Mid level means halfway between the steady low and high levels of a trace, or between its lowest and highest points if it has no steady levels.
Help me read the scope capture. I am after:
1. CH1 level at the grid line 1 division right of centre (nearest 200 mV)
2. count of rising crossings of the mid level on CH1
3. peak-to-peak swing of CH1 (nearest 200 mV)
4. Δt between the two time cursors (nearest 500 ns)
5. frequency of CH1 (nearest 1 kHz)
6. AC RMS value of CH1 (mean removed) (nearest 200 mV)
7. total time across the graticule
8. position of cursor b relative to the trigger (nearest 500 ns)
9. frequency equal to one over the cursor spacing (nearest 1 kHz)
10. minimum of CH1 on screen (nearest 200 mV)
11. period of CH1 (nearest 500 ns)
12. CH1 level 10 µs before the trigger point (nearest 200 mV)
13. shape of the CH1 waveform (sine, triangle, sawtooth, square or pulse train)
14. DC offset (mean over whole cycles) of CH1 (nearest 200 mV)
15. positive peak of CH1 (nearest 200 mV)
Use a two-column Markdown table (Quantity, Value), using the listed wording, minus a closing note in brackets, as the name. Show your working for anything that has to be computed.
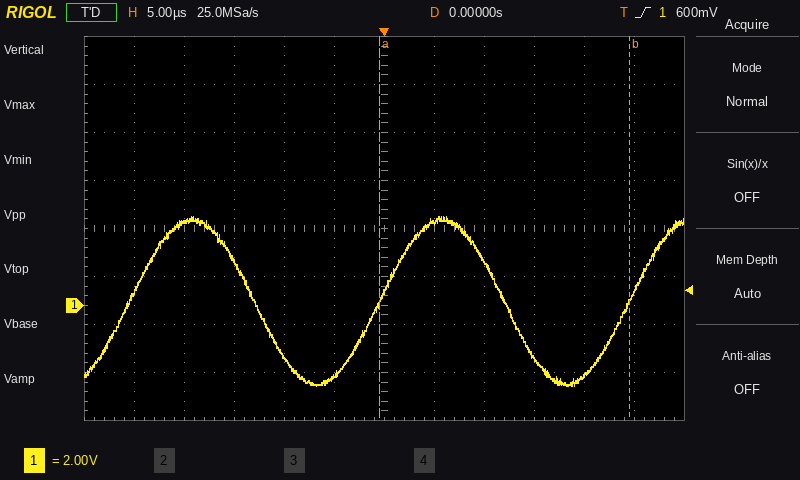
| Quantity | Value |
|---|---|
| CH1 level at the grid line 1 division right of centre | 3.4 V |
| count of rising crossings of the mid level on CH1 | 3 |
| peak-to-peak swing of CH1 | 3.6 V − (-3.4 V) = 7.0 V |
| Δt between the two time cursors | 25.0 µs |
| frequency of CH1 | 1 / 25.0 µs ≈ 40 kHz |
| AC RMS value of CH1 (mean removed) | 7.0 V / (2√2) ≈ 2.47 V, so 2.4 V to the nearest 200 mV |
| total time across the graticule | 60 µs |
| position of cursor b relative to the trigger | +24.5 µs |
| frequency equal to one over the cursor spacing | 1 / 25.0 µs ≈ 40 kHz |
| minimum of CH1 on screen | -3.4 V |
| period of CH1 | 25.0 µs |
| CH1 level 10 µs before the trigger point | -2.2 V |
| shape of the CH1 waveform | sine |
| DC offset (mean over whole cycles) of CH1 | (3.6 V + (-3.4 V)) / 2 ≈ 100 mV, so 200 mV to the nearest 200 mV |
| positive peak of CH1 | 3.6 V |
